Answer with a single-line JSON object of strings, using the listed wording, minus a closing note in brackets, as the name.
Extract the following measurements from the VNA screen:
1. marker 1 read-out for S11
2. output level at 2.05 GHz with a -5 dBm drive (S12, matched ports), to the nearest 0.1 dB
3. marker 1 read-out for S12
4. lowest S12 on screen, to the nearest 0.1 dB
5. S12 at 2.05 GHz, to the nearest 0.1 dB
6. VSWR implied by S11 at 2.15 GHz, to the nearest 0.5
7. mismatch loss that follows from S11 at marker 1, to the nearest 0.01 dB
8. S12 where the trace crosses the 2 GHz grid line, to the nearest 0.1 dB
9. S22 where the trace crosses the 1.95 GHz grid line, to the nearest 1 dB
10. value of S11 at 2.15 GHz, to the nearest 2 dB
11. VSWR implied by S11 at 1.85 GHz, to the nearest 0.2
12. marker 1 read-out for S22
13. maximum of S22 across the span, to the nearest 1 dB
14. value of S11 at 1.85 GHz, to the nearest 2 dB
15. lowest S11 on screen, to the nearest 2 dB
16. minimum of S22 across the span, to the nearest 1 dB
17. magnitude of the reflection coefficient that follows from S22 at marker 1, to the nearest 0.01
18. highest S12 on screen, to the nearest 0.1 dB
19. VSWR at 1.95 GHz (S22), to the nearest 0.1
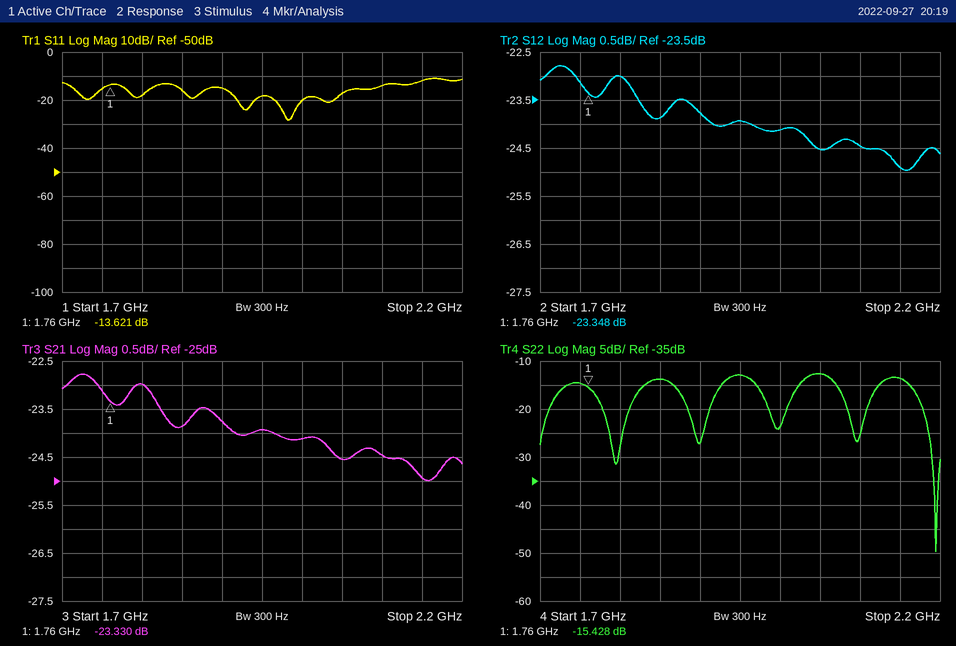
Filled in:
{"marker 1 read-out for S11": "-13.621 dB", "output level at 2.05 GHz with a -5 dBm drive (S12, matched ports), to the nearest 0.1 dB": "-29.5 dBm", "marker 1 read-out for S12": "-23.348 dB", "lowest S12 on screen, to the nearest 0.1 dB": "-25.0 dB", "S12 at 2.05 GHz, to the nearest 0.1 dB": "-24.5 dB", "VSWR implied by S11 at 2.15 GHz, to the nearest 0.5": "1.5", "mismatch loss that follows from S11 at marker 1, to the nearest 0.01 dB": "0.19 dB", "S12 where the trace crosses the 2 GHz grid line, to the nearest 0.1 dB": "-24.1 dB", "S22 where the trace crosses the 1.95 GHz grid line, to the nearest 1 dB": "-13 dB", "value of S11 at 2.15 GHz, to the nearest 2 dB": "-12 dB", "VSWR implied by S11 at 1.85 GHz, to the nearest 0.2": "1.4", "marker 1 read-out for S22": "-15.428 dB", "maximum of S22 across the span, to the nearest 1 dB": "-13 dB", "value of S11 at 1.85 GHz, to the nearest 2 dB": "-16 dB", "lowest S11 on screen, to the nearest 2 dB": "-28 dB", "minimum of S22 across the span, to the nearest 1 dB": "-50 dB", "magnitude of the reflection coefficient that follows from S22 at marker 1, to the nearest 0.01": "0.17", "highest S12 on screen, to the nearest 0.1 dB": "-22.8 dB", "VSWR at 1.95 GHz (S22), to the nearest 0.1": "1.6"}
